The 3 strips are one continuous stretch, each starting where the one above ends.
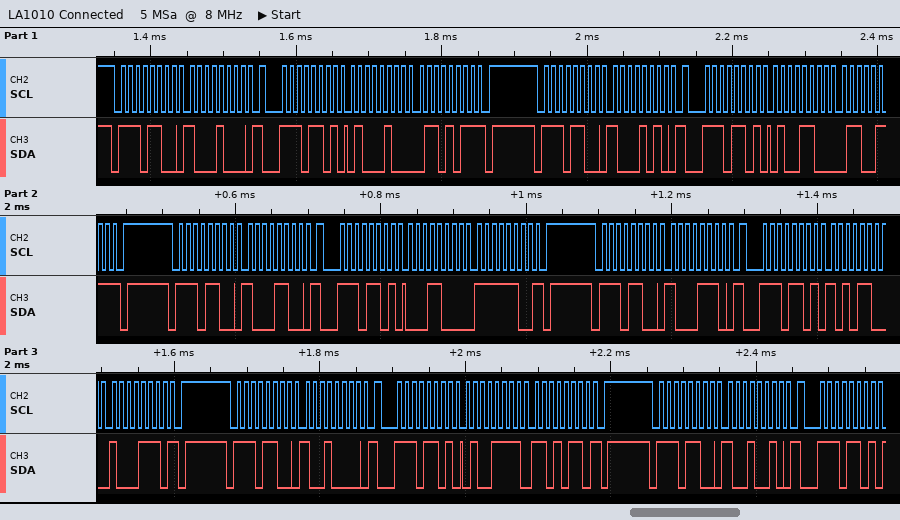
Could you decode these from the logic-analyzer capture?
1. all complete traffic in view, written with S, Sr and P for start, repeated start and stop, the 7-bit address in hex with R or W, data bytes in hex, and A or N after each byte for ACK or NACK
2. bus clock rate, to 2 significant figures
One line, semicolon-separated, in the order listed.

S 76W A 88 A Sr 76R A 44 A 6B N P S 76W A 8A A Sr 76R A 4C A 67 N P S 76W A 8C A Sr 76R A 18 A FC N P S 76W A 8E A Sr 76R A AC A 8E N P S 76W A 90 A Sr 76R A 4F A D6 N P S 76W A 92 A Sr 76R A; 100 kHz
